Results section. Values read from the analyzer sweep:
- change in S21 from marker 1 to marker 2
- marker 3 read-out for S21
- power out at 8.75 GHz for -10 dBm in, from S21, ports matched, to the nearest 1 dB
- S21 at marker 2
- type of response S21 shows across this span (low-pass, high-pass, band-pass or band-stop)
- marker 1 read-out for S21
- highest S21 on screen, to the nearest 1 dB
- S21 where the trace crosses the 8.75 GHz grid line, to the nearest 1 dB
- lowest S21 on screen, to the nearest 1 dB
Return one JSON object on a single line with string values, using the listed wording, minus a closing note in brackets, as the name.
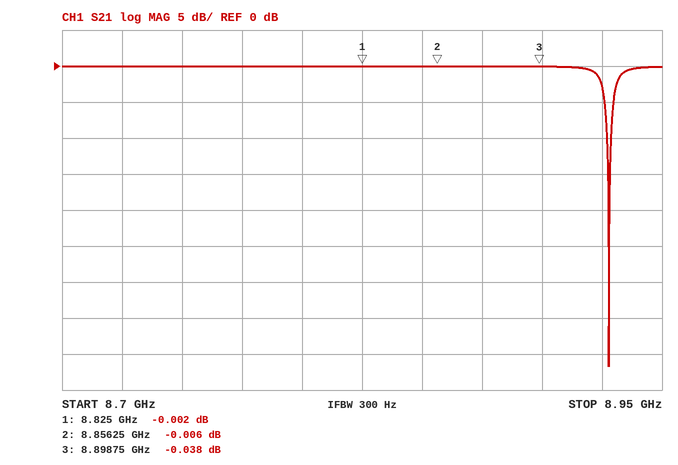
{"change in S21 from marker 1 to marker 2": "-0.004 dB", "marker 3 read-out for S21": "-0.038 dB", "power out at 8.75 GHz for -10 dBm in, from S21, ports matched, to the nearest 1 dB": "-10 dBm", "S21 at marker 2": "-0.006 dB", "type of response S21 shows across this span": "band-stop", "marker 1 read-out for S21": "-0.002 dB", "highest S21 on screen, to the nearest 1 dB": "0 dB", "S21 where the trace crosses the 8.75 GHz grid line, to the nearest 1 dB": "0 dB", "lowest S21 on screen, to the nearest 1 dB": "-42 dB"}
